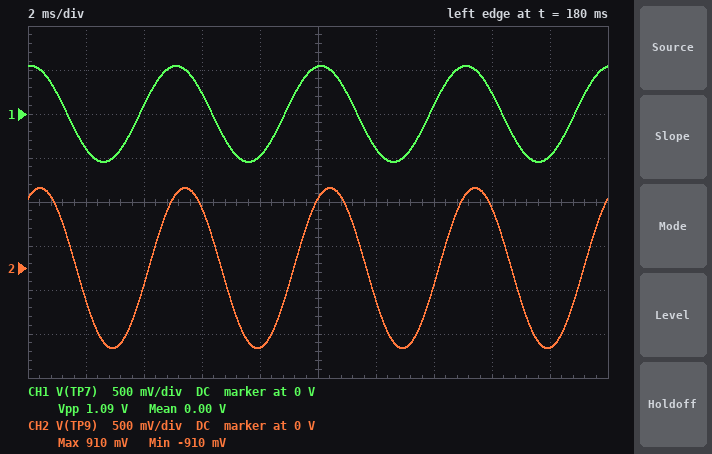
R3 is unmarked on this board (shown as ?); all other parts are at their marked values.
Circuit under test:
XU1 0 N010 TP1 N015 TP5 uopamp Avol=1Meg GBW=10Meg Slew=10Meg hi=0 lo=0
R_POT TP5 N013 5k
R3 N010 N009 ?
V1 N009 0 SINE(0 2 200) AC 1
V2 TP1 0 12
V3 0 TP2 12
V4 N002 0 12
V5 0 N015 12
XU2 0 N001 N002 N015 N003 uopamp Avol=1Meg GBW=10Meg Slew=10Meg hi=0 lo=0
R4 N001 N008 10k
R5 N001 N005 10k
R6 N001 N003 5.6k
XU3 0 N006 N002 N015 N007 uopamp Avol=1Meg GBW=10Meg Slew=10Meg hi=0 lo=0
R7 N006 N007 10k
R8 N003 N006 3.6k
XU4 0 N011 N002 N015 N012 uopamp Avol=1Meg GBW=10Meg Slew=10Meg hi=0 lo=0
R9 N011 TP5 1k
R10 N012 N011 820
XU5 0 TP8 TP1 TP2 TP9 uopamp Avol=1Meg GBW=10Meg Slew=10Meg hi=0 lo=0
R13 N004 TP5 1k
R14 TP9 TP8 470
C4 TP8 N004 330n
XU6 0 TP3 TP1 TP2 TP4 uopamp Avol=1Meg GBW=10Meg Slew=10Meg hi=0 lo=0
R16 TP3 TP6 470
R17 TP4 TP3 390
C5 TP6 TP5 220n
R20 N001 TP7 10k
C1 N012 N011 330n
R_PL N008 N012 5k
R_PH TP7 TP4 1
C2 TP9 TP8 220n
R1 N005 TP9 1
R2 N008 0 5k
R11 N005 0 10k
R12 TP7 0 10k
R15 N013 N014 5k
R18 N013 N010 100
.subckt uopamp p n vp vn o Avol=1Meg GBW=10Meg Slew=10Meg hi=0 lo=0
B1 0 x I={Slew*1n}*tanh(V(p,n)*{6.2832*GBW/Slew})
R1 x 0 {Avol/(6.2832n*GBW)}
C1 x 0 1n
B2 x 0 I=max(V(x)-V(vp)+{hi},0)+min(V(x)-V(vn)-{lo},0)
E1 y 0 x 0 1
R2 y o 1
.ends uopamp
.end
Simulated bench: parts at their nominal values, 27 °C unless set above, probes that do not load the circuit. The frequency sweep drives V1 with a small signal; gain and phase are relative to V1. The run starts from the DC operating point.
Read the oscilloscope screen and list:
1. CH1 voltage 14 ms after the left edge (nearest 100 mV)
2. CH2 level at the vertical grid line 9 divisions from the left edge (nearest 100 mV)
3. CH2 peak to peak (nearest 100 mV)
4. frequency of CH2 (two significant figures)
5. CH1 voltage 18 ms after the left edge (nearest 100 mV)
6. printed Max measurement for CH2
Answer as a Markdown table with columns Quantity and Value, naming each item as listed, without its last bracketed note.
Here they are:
| Quantity | Value |
|---|---|
| CH1 voltage 14 ms after the left edge | 100 mV |
| CH2 level at the vertical grid line 9 divisions from the left edge | -900 mV |
| CH2 peak to peak | 1.8 V |
| frequency of CH2 | 200 Hz |
| CH1 voltage 18 ms after the left edge | -500 mV |
| printed Max measurement for CH2 | 910 mV |
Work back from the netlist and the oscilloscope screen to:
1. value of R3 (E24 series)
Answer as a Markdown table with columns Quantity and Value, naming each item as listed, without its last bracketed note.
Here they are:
| Quantity | Value |
|---|---|
| value of R3 | 2 kΩ |
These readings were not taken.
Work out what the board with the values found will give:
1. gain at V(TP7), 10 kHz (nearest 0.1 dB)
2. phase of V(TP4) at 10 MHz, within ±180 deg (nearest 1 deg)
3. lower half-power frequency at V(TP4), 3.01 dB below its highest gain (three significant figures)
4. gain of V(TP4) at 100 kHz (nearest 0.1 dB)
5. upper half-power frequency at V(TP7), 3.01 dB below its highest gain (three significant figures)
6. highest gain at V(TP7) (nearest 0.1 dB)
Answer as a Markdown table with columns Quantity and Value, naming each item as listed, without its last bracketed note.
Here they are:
| Quantity | Value |
|---|---|
| gain at V(TP7), 10 kHz | 6.4 dB |
| phase of V(TP4) at 10 MHz, within ±180 deg | -136 deg |
| lower half-power frequency at V(TP4), 3.01 dB below its highest gain | 1.54 kHz |
| gain of V(TP4) at 100 kHz | 6.5 dB |
| upper half-power frequency at V(TP7), 3.01 dB below its highest gain | 2.33 MHz |
| highest gain at V(TP7) | 6.5 dB |
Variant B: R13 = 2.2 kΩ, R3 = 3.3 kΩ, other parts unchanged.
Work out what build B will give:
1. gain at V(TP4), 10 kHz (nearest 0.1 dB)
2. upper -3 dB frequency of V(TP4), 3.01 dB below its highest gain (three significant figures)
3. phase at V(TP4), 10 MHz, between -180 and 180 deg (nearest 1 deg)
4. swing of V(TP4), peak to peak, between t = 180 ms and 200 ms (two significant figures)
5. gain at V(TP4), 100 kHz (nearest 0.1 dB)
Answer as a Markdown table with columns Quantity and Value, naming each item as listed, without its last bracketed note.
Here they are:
| Quantity | Value |
|---|---|
| gain at V(TP4), 10 kHz | 2.1 dB |
| upper -3 dB frequency of V(TP4), 3.01 dB below its highest gain | 2.92 MHz |
| phase at V(TP4), 10 MHz, between -180 and 180 deg | -130 deg |
| swing of V(TP4), peak to peak, between t = 180 ms and 200 ms | 660 mV |
| gain at V(TP4), 100 kHz | 2.2 dB |
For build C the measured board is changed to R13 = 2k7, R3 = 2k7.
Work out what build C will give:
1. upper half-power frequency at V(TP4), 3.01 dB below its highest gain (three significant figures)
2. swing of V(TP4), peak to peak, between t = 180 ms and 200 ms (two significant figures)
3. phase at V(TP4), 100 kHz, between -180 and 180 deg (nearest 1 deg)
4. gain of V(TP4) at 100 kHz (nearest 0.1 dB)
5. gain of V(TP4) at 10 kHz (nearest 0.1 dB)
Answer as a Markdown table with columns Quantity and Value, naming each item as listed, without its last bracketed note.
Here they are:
| Quantity | Value |
|---|---|
| upper half-power frequency at V(TP4), 3.01 dB below its highest gain | 2.69 MHz |
| swing of V(TP4), peak to peak, between t = 180 ms and 200 ms | 810 mV |
| phase at V(TP4), 100 kHz, between -180 and 180 deg | -2 deg |
| gain of V(TP4) at 100 kHz | 3.9 dB |
| gain of V(TP4) at 10 kHz | 3.8 dB |
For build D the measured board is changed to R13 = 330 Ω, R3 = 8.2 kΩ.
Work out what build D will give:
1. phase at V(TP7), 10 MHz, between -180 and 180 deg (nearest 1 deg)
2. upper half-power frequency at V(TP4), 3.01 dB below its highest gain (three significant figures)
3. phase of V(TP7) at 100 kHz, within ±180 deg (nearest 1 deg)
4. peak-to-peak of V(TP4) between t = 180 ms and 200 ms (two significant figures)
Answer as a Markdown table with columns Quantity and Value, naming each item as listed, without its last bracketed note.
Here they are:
| Quantity | Value |
|---|---|
| phase at V(TP7), 10 MHz, between -180 and 180 deg | -120 deg |
| upper half-power frequency at V(TP4), 3.01 dB below its highest gain | 3.71 MHz |
| phase of V(TP7) at 100 kHz, within ±180 deg | -1 deg |
| peak-to-peak of V(TP4) between t = 180 ms and 200 ms | 270 mV |
